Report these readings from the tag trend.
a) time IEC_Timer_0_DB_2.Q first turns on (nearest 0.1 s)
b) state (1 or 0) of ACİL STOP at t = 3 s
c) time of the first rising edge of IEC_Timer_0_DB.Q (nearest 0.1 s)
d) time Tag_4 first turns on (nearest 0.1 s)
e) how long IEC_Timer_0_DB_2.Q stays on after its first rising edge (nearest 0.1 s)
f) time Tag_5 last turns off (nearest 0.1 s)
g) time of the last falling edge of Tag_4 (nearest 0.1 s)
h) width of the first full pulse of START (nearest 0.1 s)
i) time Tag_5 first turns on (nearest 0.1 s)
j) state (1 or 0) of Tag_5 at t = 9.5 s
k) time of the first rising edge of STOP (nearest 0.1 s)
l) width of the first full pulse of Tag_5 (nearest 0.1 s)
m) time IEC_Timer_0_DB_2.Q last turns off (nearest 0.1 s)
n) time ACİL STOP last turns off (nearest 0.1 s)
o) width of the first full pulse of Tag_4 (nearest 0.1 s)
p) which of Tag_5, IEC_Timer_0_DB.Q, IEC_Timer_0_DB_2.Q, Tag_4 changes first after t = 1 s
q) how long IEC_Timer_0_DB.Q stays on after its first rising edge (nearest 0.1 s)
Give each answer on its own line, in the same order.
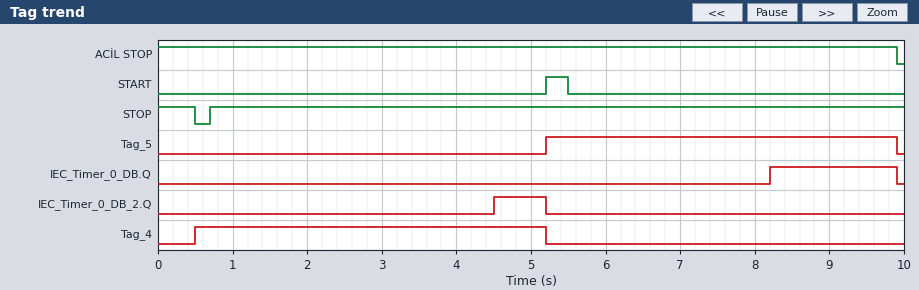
4.5 s
1
8.2 s
0.5 s
0.7 s
9.9 s
5.2 s
0.3 s
5.2 s
1
0.7 s
4.7 s
5.2 s
9.9 s
4.7 s
IEC_Timer_0_DB_2.Q
1.7 s
